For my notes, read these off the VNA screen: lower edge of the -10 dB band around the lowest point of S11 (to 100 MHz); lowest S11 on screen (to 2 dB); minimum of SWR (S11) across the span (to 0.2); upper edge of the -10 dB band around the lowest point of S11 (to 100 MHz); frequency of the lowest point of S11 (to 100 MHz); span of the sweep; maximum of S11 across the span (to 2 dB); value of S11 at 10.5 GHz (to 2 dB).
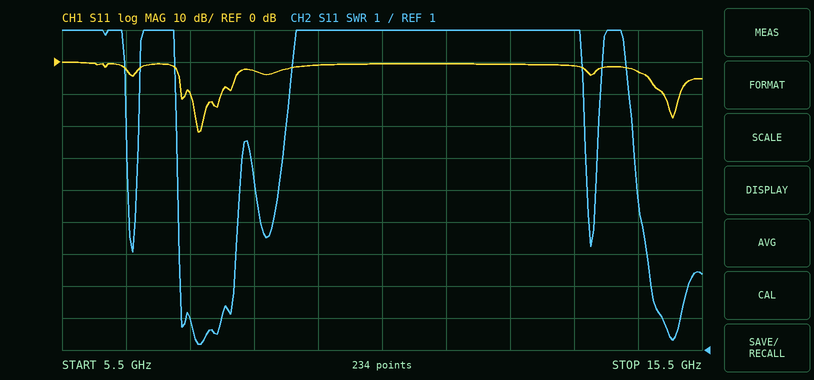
7.5 GHz
-22 dB
1.2
8.0 GHz
7.6 GHz
10 GHz
0 dB
0 dB
